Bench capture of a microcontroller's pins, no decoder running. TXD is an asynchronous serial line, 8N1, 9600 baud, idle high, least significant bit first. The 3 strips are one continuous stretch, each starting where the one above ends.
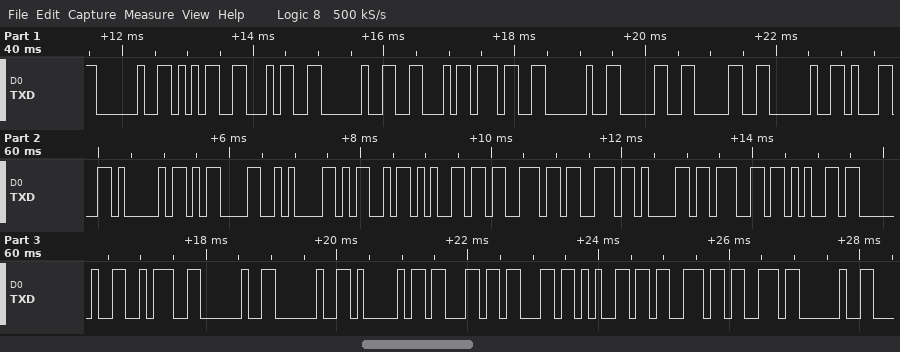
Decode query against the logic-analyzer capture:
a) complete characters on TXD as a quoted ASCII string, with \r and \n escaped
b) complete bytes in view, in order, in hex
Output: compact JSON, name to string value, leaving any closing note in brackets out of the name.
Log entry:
{"complete characters on TXD as a quoted ASCII string, with \\r and \\n escaped": "\" 54 F7 00 1A\\r\\nMessage :  Access \"", "complete bytes in view, in order, in hex": "20 35 34 20 46 37 20 30 30 20 31 41 0D 0A 4D 65 73 73 61 67 65 20 3A 20 20 41 63 63 65 73 73 20"}
